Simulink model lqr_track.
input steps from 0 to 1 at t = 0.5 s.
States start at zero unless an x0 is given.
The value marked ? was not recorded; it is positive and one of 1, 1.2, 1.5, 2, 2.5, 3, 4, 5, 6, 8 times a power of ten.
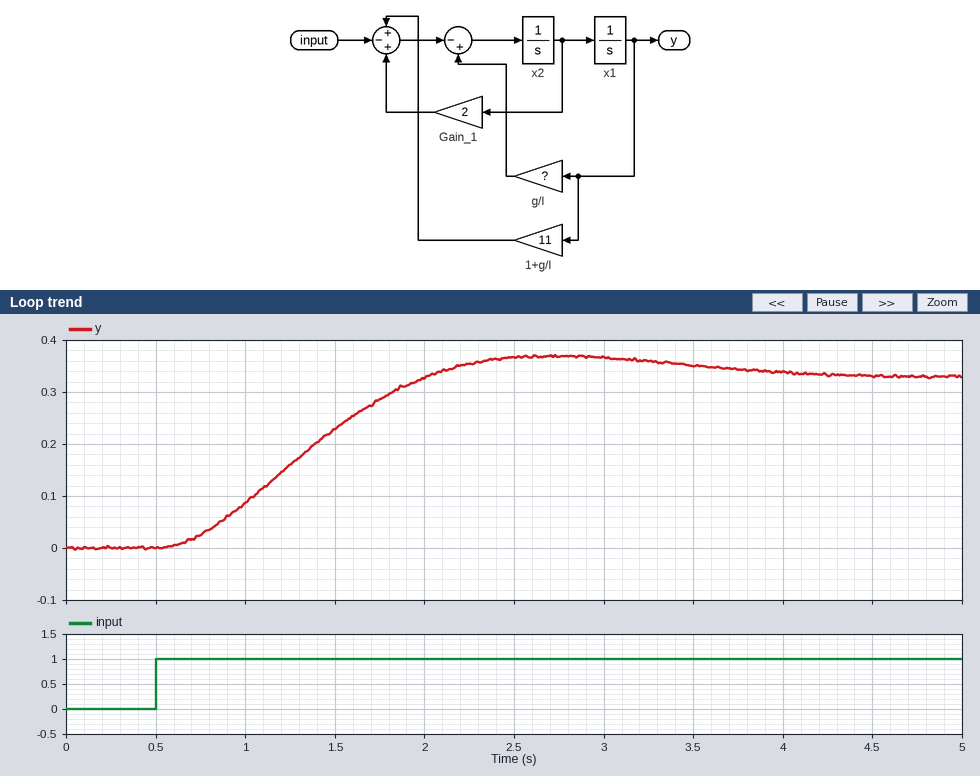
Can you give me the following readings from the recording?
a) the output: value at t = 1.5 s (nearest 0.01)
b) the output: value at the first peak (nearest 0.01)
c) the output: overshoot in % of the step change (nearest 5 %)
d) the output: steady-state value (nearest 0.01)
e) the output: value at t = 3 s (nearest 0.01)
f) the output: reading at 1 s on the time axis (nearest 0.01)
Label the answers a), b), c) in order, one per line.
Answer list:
a) 0.23
b) 0.37
c) 10 %
d) 0.33
e) 0.37
f) 0.09
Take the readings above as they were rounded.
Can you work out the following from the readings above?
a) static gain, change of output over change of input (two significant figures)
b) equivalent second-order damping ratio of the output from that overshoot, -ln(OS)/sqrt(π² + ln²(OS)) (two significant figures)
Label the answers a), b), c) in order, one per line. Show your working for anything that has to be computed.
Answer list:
a) (0.33 - 0) / (1 - 0) = 0.33
b) ln(0.1) = -2.303; 2.303 / sqrt(9.870 + 5.302) = 0.59
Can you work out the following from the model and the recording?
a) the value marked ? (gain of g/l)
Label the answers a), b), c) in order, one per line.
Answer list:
a) 8
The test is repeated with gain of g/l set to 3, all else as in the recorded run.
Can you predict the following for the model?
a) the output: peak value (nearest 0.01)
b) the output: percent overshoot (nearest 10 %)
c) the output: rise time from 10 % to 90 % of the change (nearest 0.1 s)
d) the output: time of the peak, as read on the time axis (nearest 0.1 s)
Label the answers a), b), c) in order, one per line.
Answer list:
a) 0.16
b) 30 %
c) 0.5 s
d) 1.7 s
